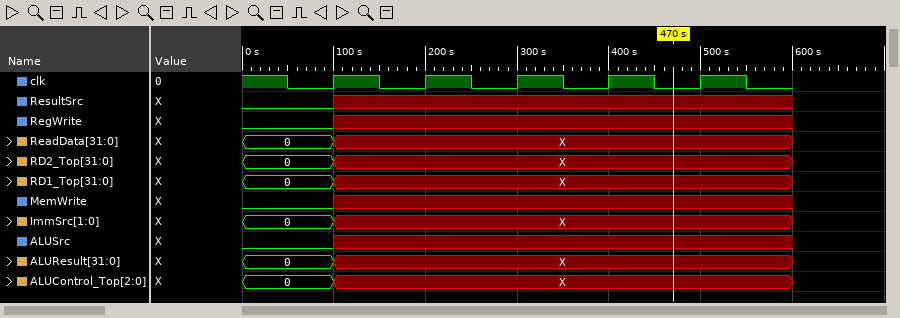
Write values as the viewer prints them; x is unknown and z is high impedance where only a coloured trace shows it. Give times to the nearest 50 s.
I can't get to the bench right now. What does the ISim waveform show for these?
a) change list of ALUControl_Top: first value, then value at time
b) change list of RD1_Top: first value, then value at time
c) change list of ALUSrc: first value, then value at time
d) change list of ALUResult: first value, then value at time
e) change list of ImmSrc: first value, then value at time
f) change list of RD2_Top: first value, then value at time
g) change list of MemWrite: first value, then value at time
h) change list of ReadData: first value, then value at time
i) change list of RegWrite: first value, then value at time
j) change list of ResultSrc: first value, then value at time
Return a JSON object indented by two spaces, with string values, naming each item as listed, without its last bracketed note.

{
  "change list of ALUControl_Top: first value, then value at time": "0, X at 100 s",
  "change list of RD1_Top: first value, then value at time": "0, X at 100 s",
  "change list of ALUSrc: first value, then value at time": "0, x at 100 s",
  "change list of ALUResult: first value, then value at time": "0, X at 100 s",
  "change list of ImmSrc: first value, then value at time": "0, X at 100 s",
  "change list of RD2_Top: first value, then value at time": "0, X at 100 s",
  "change list of MemWrite: first value, then value at time": "0, x at 100 s",
  "change list of ReadData: first value, then value at time": "0, X at 100 s",
  "change list of RegWrite: first value, then value at time": "0, x at 100 s",
  "change list of ResultSrc: first value, then value at time": "0, x at 100 s"
}
